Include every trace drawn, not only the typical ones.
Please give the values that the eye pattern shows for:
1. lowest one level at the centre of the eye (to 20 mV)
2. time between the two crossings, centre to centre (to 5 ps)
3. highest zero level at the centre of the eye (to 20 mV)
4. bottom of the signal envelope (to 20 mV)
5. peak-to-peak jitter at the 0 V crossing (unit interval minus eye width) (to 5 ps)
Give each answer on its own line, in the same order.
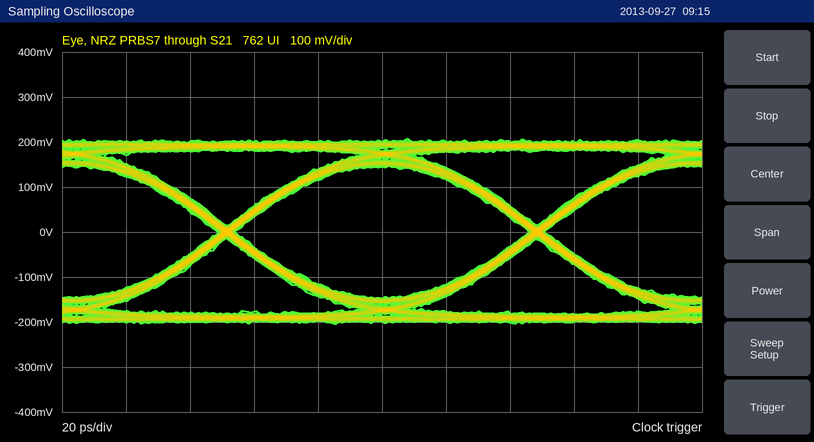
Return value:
140 mV
95 ps
-140 mV
-200 mV
5 ps
